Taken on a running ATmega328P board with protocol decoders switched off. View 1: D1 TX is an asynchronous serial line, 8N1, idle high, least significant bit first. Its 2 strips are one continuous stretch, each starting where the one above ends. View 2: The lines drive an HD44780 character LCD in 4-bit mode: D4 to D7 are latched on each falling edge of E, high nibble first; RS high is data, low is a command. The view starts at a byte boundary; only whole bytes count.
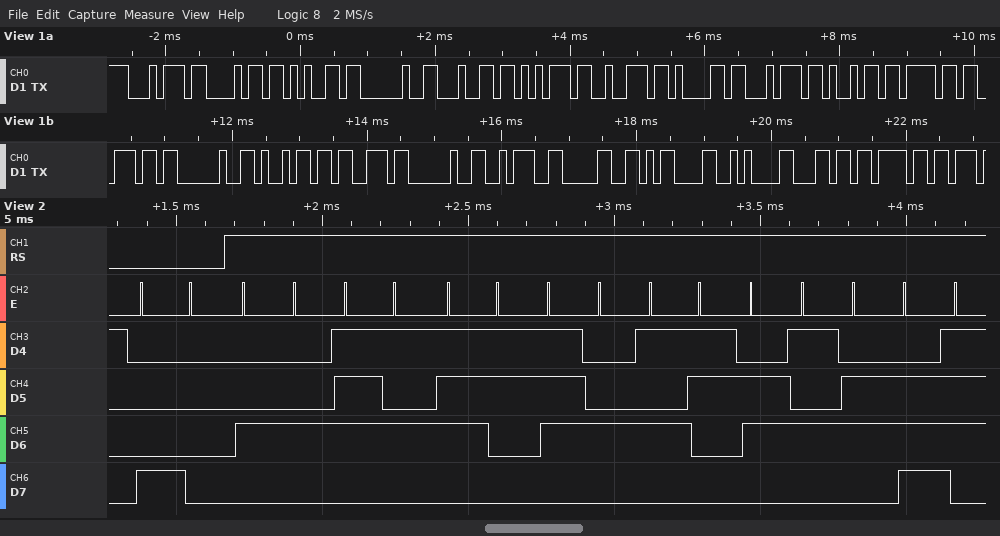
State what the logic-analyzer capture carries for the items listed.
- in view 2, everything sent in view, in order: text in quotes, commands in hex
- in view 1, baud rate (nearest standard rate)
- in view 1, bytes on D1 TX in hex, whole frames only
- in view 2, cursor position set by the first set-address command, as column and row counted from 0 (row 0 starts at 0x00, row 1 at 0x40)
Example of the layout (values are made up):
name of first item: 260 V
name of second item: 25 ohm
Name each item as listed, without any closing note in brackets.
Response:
in view 2, everything sent in view, in order: text in quotes, commands in hex: 0x80 "DustSen"
in view 1, baud rate: 9600 baud
in view 1, bytes on D1 TX in hex, whole frames only: 74 68 65 20 64 75 72 61 74 69 6F 6E 20 69 73 20 3A 30 0D 0A 6C 6F
in view 2, cursor position set by the first set-address command, as column and row counted from 0: column 0, row 0
